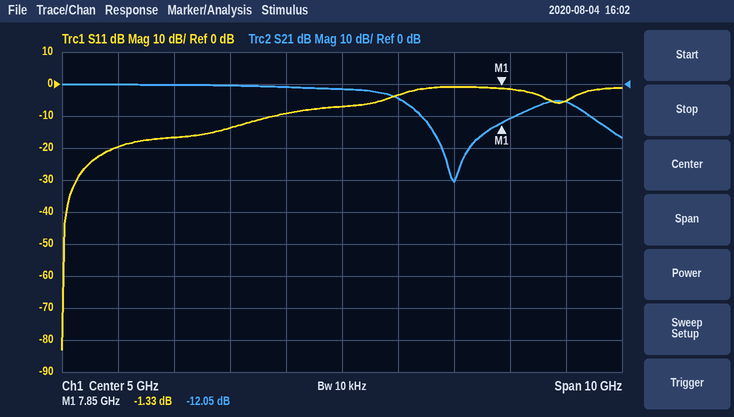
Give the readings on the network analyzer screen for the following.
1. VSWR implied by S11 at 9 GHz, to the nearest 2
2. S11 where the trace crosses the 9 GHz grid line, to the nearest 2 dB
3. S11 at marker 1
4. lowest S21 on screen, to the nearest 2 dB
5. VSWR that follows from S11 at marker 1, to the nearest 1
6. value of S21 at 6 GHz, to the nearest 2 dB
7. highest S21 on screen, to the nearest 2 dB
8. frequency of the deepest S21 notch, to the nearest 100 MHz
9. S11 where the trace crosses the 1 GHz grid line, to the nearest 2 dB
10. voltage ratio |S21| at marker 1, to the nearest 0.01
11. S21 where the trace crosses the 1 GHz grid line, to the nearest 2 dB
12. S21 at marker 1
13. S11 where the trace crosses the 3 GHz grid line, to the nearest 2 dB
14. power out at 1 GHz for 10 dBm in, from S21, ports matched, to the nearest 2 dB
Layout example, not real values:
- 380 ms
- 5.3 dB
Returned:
- 4
- -6 dB
- -1.33 dB
- -30 dB
- 13
- -4 dB
- 0 dB
- 7.0 GHz
- -20 dB
- 0.25
- 0 dB
- -12.05 dB
- -14 dB
- 10 dBm
